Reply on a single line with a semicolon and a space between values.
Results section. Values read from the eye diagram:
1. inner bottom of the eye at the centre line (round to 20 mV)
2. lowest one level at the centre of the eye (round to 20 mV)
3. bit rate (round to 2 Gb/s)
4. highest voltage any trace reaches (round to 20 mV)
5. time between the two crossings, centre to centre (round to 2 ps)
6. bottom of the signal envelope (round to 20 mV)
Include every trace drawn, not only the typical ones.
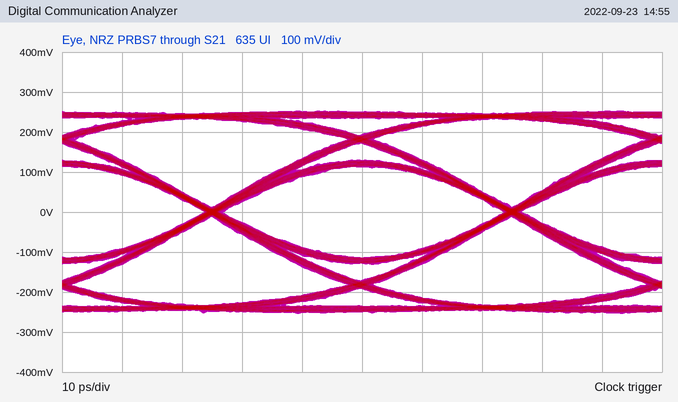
-120 mV; 120 mV; 20 Gb/s; 260 mV; 50 ps; -260 mV
